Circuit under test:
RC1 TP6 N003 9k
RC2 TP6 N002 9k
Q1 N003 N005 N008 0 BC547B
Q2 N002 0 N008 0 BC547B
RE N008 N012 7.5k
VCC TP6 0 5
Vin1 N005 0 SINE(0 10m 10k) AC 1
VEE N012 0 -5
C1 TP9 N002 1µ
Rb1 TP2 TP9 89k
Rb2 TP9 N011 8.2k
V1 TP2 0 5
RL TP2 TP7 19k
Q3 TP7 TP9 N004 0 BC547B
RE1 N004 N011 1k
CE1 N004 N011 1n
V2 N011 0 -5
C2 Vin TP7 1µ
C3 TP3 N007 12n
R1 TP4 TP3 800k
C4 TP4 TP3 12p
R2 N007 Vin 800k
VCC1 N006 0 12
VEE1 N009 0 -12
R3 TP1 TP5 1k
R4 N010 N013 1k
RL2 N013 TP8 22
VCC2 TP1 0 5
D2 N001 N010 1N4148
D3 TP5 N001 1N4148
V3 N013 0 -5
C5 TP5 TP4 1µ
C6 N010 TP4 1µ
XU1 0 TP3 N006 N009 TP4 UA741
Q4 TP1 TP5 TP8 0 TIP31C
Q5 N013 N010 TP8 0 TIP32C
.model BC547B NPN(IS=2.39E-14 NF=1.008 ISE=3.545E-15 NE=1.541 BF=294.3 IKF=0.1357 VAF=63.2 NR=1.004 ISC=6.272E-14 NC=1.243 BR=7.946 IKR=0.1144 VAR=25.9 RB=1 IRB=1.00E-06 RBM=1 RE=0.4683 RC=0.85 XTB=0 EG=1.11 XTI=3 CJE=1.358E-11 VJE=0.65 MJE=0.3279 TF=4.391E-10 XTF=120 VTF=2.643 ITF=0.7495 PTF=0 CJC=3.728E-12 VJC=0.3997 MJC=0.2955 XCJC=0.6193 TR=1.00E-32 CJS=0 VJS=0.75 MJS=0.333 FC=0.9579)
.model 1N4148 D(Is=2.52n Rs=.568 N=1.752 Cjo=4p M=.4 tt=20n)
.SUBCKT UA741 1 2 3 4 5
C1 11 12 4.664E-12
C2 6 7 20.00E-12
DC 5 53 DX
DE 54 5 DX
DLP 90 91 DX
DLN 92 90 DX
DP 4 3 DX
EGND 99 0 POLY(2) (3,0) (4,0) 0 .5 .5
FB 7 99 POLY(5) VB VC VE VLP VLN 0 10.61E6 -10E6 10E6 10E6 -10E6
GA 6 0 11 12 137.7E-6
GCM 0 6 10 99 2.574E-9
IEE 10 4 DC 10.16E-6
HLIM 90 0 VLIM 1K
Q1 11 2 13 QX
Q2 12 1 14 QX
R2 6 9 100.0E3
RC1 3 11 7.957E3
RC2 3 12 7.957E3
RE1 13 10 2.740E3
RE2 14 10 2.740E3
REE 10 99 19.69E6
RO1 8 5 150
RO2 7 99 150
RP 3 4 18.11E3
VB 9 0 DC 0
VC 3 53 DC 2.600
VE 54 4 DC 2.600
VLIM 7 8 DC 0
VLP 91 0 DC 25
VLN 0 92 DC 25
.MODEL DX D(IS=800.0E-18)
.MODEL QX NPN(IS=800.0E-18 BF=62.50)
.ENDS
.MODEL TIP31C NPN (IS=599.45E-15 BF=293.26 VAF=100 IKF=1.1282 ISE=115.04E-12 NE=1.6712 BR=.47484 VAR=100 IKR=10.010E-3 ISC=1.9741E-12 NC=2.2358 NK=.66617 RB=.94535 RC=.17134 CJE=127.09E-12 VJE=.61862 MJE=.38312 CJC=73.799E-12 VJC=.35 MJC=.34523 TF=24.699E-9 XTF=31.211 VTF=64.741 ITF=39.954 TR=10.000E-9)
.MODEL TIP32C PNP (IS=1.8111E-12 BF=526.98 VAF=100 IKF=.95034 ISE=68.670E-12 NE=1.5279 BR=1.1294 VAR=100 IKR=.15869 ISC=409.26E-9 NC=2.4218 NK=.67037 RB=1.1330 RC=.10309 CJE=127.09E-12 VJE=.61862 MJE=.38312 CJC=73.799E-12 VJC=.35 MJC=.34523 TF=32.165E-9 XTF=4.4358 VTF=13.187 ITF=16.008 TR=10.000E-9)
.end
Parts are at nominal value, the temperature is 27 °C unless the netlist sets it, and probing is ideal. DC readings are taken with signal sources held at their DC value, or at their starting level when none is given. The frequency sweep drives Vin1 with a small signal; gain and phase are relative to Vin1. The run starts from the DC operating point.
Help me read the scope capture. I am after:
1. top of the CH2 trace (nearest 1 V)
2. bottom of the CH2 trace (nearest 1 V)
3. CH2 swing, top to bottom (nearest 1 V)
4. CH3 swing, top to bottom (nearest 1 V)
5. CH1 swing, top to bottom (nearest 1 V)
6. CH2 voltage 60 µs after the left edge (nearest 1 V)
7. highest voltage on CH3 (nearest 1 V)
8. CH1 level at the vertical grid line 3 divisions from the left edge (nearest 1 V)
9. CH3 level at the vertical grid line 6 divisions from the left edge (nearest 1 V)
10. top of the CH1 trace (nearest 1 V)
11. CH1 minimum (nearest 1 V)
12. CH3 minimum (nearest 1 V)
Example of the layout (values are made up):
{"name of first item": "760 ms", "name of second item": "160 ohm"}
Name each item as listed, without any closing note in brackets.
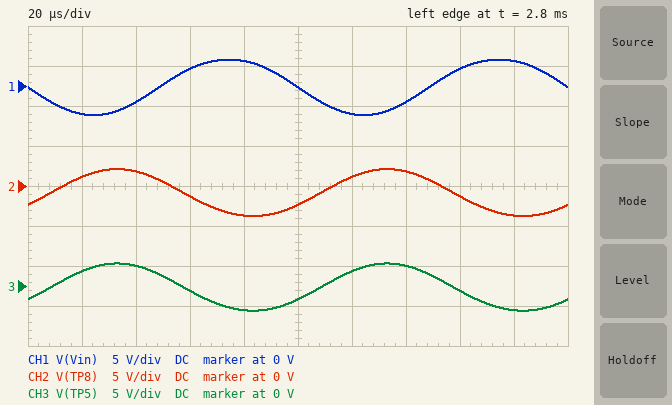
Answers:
{"top of the CH2 trace": "2 V", "bottom of the CH2 trace": "-4 V", "CH2 swing, top to bottom": "6 V", "CH3 swing, top to bottom": "6 V", "CH1 swing, top to bottom": "7 V", "CH2 voltage 60 µs after the left edge": "-1 V", "highest voltage on CH3": "3 V", "CH1 level at the vertical grid line 3 divisions from the left edge": "2 V", "CH3 level at the vertical grid line 6 divisions from the left edge": "2 V", "top of the CH1 trace": "3 V", "CH1 minimum": "-4 V", "CH3 minimum": "-3 V"}
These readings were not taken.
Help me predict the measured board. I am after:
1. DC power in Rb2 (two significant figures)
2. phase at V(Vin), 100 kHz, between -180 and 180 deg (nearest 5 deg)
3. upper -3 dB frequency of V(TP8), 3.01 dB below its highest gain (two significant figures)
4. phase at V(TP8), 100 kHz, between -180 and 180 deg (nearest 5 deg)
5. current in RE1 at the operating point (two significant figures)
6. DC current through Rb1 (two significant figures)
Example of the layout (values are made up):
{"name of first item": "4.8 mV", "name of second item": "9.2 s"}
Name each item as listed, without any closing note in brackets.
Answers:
{"DC power in Rb2": "86 µW", "phase at V(Vin), 100 kHz, between -180 and 180 deg": "-160 deg", "upper -3 dB frequency of V(TP8), 3.01 dB below its highest gain": "17 kHz", "phase at V(TP8), 100 kHz, between -180 and 180 deg": "-65 deg", "current in RE1 at the operating point": "240 µA", "DC current through Rb1": "100 µA"}
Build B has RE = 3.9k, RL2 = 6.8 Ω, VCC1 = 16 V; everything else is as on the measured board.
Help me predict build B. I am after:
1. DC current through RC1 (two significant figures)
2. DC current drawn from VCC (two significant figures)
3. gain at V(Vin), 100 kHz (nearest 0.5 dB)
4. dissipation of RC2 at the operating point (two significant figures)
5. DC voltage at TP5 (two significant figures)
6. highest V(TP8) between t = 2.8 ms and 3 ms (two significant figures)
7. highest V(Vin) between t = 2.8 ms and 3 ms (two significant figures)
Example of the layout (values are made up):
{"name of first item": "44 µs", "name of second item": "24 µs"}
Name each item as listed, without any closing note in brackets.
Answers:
{"DC current through RC1": "560 µA", "DC current drawn from VCC": "1.1 mA", "gain at V(Vin), 100 kHz": "58.0 dB", "dissipation of RC2 at the operating point": "2.8 mW", "DC voltage at TP5": "-1.4 V", "highest V(TP8) between t = 2.8 ms and 3 ms": "2.2 V", "highest V(Vin) between t = 2.8 ms and 3 ms": "4.4 V"}
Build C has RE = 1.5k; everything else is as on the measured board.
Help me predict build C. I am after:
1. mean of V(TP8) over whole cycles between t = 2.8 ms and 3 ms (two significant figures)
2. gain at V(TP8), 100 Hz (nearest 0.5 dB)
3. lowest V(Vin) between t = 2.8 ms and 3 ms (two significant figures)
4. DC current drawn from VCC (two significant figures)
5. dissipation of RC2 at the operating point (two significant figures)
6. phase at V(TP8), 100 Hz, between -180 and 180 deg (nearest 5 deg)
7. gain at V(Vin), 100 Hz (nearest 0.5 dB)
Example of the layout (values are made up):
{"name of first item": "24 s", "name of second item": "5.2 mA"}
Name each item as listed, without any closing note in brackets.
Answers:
{"mean of V(TP8) over whole cycles between t = 2.8 ms and 3 ms": "-860 mV", "gain at V(TP8), 100 Hz": "11.5 dB", "lowest V(Vin) between t = 2.8 ms and 3 ms": "-95 mV", "DC current drawn from VCC": "1.3 mA", "dissipation of RC2 at the operating point": "3.6 mW", "phase at V(TP8), 100 Hz, between -180 and 180 deg": "85 deg", "gain at V(Vin), 100 Hz": "18.5 dB"}
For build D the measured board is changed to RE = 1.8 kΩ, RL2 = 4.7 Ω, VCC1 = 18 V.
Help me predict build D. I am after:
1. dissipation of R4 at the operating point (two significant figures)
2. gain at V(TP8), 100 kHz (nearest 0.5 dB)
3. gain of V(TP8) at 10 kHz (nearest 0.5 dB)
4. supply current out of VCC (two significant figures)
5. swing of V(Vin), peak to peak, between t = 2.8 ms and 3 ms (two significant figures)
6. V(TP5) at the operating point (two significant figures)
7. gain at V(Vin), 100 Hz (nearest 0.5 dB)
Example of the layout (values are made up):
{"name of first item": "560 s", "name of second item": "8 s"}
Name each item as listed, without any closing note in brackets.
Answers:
{"dissipation of R4 at the operating point": "3.6 mW", "gain at V(TP8), 100 kHz": "4.5 dB", "gain of V(TP8) at 10 kHz": "17.5 dB", "supply current out of VCC": "1.3 mA", "swing of V(Vin), peak to peak, between t = 2.8 ms and 3 ms": "180 mV", "V(TP5) at the operating point": "-1.9 V", "gain at V(Vin), 100 Hz": "19.0 dB"}
